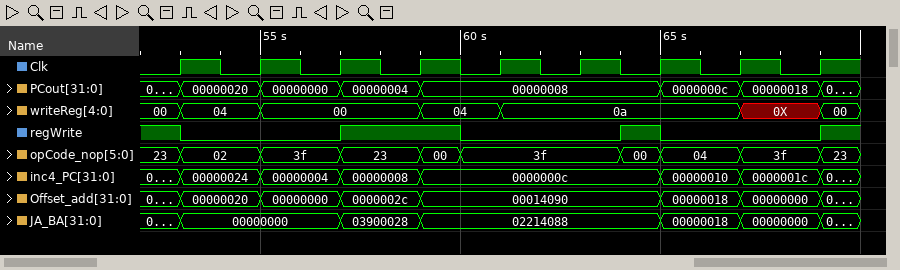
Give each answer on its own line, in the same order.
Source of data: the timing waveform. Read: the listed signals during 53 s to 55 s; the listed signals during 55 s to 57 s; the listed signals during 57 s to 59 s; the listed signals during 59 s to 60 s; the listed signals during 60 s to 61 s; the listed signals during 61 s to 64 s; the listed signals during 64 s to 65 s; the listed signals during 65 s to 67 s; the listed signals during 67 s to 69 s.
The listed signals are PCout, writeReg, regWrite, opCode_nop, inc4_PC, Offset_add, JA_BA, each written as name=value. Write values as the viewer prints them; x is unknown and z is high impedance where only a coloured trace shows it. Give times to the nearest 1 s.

PCout=00000020, writeReg=04, regWrite=0, opCode_nop=02, inc4_PC=00000024, Offset_add=00000020, JA_BA=00000000
PCout=00000000, writeReg=00, regWrite=0, opCode_nop=3f, inc4_PC=00000004, Offset_add=00000000, JA_BA=00000000
PCout=00000004, writeReg=00, regWrite=1, opCode_nop=23, inc4_PC=00000008, Offset_add=0000002c, JA_BA=03900028
PCout=00000008, writeReg=04, regWrite=1, opCode_nop=00, inc4_PC=0000000c, Offset_add=00014090, JA_BA=02214088
PCout=00000008, writeReg=04, regWrite=0, opCode_nop=3f, inc4_PC=0000000c, Offset_add=00014090, JA_BA=02214088
PCout=00000008, writeReg=0a, regWrite=0, opCode_nop=3f, inc4_PC=0000000c, Offset_add=00014090, JA_BA=02214088
PCout=00000008, writeReg=0a, regWrite=1, opCode_nop=00, inc4_PC=0000000c, Offset_add=00014090, JA_BA=02214088
PCout=0000000c, writeReg=0a, regWrite=0, opCode_nop=04, inc4_PC=00000010, Offset_add=00000018, JA_BA=00000018
PCout=00000018, writeReg=0X, regWrite=0, opCode_nop=3f, inc4_PC=0000001c, Offset_add=00000000, JA_BA=00000000
